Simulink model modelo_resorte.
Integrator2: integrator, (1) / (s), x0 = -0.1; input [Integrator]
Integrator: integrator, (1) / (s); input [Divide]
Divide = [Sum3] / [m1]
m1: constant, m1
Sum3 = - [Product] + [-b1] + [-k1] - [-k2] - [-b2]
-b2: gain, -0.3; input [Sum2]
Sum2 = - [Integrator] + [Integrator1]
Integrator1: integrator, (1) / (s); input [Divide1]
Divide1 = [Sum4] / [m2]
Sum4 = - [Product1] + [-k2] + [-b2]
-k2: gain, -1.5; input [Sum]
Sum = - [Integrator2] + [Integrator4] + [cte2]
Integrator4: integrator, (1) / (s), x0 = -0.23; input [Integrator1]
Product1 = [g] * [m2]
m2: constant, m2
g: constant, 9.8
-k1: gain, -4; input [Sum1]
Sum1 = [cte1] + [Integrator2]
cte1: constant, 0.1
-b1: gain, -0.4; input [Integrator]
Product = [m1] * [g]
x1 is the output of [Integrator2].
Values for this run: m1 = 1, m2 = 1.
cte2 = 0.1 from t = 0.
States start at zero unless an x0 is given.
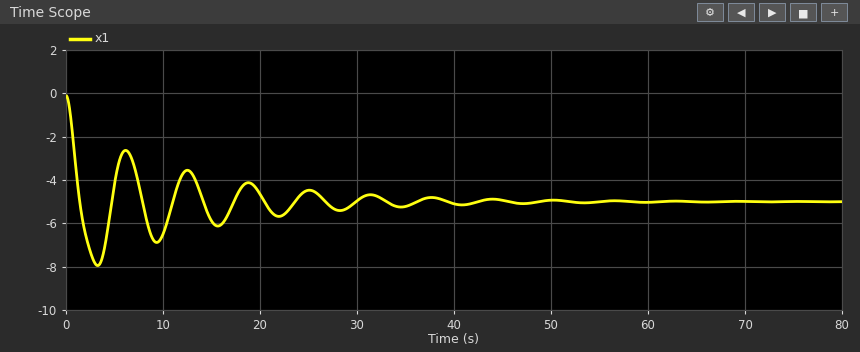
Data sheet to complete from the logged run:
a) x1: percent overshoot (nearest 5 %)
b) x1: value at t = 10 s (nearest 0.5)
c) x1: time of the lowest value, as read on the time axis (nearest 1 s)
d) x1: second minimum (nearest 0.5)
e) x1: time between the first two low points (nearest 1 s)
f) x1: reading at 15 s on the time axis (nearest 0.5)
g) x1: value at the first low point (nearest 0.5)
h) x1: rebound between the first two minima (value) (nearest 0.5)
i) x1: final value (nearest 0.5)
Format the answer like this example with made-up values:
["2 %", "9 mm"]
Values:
["60 %", "-6.5", "3 s", "-7.0", "6 s", "-6.0", "-8.0", "-2.5", "-5.0"]
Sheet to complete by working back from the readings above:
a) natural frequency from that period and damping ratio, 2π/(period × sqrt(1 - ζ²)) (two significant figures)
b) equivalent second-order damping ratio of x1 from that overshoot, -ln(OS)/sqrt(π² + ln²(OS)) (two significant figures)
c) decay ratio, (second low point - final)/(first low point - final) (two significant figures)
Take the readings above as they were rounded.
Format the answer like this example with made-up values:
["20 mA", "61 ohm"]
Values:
["1.1 rad/s", "0.16", "0.67"]
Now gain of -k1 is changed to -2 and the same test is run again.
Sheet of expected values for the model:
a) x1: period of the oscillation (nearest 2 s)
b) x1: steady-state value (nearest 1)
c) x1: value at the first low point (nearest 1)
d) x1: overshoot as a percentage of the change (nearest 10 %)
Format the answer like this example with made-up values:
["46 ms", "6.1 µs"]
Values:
["8 s", "-10", "-17", "70 %"]
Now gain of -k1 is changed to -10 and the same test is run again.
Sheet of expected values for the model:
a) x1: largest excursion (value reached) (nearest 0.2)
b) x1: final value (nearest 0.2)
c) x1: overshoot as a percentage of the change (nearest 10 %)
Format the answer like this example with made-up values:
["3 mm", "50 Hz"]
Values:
["-3.2", "-2.0", "60 %"]
